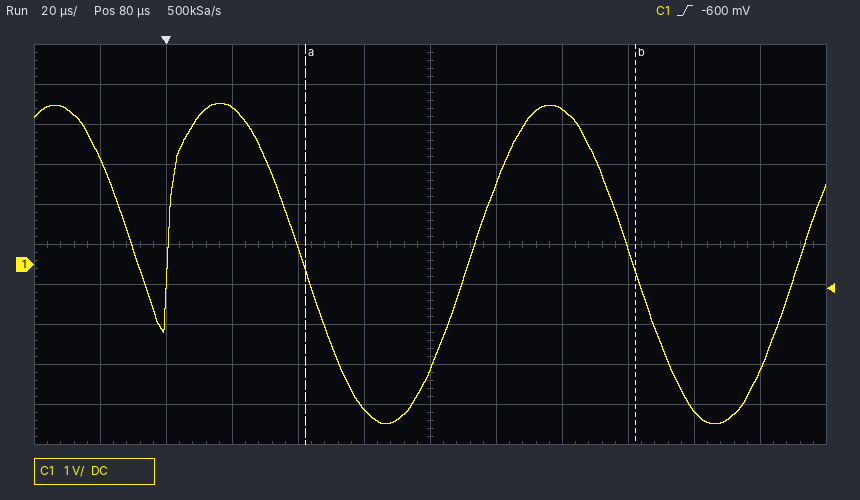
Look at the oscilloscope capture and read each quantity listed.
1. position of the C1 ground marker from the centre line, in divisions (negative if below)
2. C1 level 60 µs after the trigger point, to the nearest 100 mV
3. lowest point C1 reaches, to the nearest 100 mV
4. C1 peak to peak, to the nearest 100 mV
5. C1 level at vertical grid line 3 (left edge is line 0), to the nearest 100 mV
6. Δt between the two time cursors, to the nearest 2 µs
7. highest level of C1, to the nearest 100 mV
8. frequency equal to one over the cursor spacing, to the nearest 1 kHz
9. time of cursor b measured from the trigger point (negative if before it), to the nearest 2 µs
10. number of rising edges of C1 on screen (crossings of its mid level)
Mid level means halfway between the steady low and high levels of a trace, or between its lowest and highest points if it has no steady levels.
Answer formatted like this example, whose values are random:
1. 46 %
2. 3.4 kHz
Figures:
1. -0.5 div
2. -3.6 V
3. -4.0 V
4. 8.0 V
5. 3.9 V
6. 100 µs
7. 4.0 V
8. 10 kHz
9. +142 µs
10. 3
